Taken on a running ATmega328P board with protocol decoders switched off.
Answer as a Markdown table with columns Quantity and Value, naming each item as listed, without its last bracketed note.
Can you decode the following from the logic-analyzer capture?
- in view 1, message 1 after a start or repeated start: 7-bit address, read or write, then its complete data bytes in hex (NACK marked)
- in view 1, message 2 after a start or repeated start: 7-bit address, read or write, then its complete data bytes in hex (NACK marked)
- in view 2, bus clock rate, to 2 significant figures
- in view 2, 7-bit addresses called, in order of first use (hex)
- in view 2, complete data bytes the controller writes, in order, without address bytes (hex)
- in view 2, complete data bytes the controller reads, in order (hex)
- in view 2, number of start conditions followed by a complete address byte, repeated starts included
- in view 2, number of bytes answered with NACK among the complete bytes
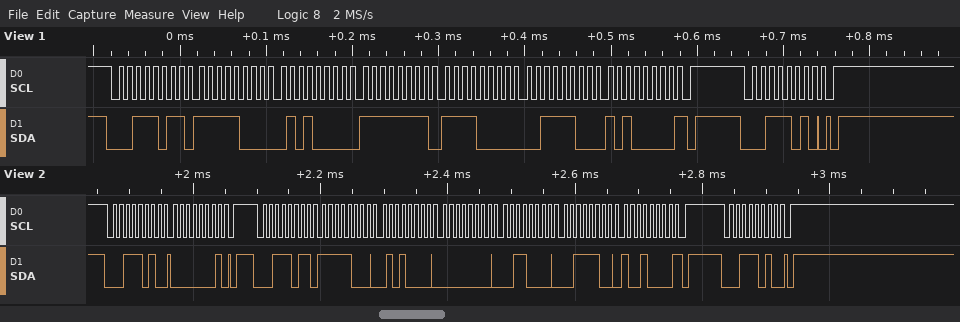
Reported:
| Quantity | Value |
|---|---|
| in view 1, message 1 after a start or repeated start: 7-bit address, read or write, then its complete data bytes in hex | 0x1D read: F8 50 FF F0 3C A0 NACK |
| in view 1, message 2 after a start or repeated start: 7-bit address, read or write, then its complete data bytes in hex | 0x1D write |
| in view 2, bus clock rate, to 2 significant figures | 100 kHz |
| in view 2, 7-bit addresses called, in order of first use | 0x1D |
| in view 2, complete data bytes the controller writes, in order, without address bytes | 01 |
| in view 2, complete data bytes the controller reads, in order | F8 50 00 30 3C 90 |
| in view 2, number of start conditions followed by a complete address byte, repeated starts included | 3 |
| in view 2, number of bytes answered with NACK among the complete bytes | 1 |
